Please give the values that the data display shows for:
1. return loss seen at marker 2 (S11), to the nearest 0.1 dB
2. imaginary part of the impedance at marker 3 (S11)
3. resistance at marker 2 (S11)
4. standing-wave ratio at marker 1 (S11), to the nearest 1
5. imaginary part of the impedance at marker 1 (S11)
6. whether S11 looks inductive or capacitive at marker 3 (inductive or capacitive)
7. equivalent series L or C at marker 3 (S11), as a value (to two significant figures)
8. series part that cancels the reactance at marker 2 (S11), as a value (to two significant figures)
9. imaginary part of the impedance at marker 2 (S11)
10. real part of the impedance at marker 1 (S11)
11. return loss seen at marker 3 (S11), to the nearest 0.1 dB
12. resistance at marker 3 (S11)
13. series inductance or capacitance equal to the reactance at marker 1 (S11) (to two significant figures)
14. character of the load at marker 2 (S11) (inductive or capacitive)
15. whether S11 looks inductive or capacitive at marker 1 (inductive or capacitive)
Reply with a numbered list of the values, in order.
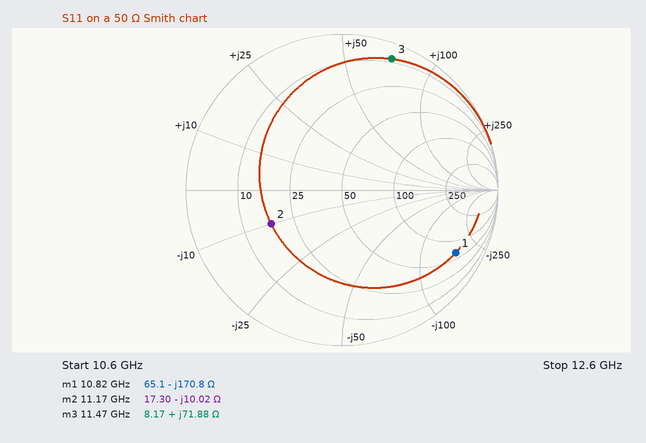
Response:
1. 6.0 dB
2. +71.88 Ω
3. 17.30 Ω
4. 11
5. -170.8 Ω
6. inductive
7. 1.00 nH
8. 140 pH
9. -10.02 Ω
10. 65.1 Ω
11. 0.9 dB
12. 8.17 Ω
13. 86 fF
14. capacitive
15. capacitive
